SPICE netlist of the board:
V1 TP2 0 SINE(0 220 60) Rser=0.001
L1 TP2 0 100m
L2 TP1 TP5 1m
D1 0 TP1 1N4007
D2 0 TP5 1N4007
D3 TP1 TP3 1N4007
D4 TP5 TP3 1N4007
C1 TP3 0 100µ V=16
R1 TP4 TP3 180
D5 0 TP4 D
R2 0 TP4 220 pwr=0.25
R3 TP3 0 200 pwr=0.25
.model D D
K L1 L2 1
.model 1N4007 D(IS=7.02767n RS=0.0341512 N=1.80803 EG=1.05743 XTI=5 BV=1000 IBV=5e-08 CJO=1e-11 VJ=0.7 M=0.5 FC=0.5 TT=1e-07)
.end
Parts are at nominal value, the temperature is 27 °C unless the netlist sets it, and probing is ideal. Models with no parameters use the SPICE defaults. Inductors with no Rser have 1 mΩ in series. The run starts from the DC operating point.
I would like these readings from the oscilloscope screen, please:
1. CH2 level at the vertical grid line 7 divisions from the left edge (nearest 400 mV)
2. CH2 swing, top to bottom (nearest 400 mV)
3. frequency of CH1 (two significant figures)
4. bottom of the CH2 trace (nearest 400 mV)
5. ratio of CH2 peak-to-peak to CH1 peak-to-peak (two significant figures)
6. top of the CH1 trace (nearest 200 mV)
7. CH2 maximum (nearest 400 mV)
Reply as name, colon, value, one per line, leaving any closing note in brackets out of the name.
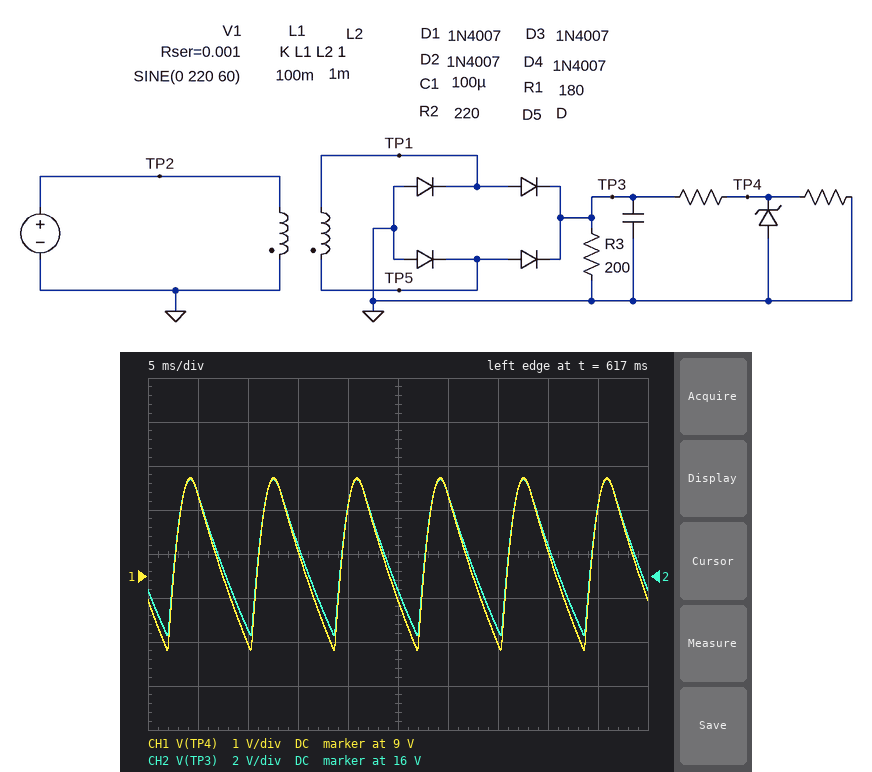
CH2 level at the vertical grid line 7 divisions from the left edge: 13.6 V
CH2 swing, top to bottom: 7.2 V
frequency of CH1: 120 Hz
bottom of the CH2 trace: 13.2 V
ratio of CH2 peak-to-peak to CH1 peak-to-peak: 1.8
top of the CH1 trace: 11.2 V
CH2 maximum: 20.4 V
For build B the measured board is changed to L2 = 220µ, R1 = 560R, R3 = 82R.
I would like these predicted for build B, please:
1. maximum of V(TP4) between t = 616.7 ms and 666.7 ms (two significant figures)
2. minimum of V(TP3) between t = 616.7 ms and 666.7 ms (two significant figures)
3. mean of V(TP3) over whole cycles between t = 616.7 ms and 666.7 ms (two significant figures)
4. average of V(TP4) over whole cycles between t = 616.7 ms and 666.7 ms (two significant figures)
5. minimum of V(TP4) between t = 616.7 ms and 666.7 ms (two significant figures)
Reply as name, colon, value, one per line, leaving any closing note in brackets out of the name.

maximum of V(TP4) between t = 616.7 ms and 666.7 ms: 2.5 V
minimum of V(TP3) between t = 616.7 ms and 666.7 ms: 4.4 V
mean of V(TP3) over whole cycles between t = 616.7 ms and 666.7 ms: 6.7 V
average of V(TP4) over whole cycles between t = 616.7 ms and 666.7 ms: 1.9 V
minimum of V(TP4) between t = 616.7 ms and 666.7 ms: 1.2 V
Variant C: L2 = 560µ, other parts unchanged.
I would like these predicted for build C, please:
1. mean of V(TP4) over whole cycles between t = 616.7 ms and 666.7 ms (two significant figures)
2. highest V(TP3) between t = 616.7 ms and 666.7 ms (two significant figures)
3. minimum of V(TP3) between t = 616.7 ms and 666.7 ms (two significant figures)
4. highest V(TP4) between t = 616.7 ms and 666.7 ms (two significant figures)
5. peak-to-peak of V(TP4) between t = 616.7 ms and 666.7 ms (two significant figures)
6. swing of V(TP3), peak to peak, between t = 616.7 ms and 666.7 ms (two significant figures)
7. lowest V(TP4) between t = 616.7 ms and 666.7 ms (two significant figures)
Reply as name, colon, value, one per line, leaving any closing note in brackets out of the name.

mean of V(TP4) over whole cycles between t = 616.7 ms and 666.7 ms: 6.9 V
highest V(TP3) between t = 616.7 ms and 666.7 ms: 15 V
minimum of V(TP3) between t = 616.7 ms and 666.7 ms: 9.7 V
highest V(TP4) between t = 616.7 ms and 666.7 ms: 8.2 V
peak-to-peak of V(TP4) between t = 616.7 ms and 666.7 ms: 2.9 V
swing of V(TP3), peak to peak, between t = 616.7 ms and 666.7 ms: 5.2 V
lowest V(TP4) between t = 616.7 ms and 666.7 ms: 5.3 V
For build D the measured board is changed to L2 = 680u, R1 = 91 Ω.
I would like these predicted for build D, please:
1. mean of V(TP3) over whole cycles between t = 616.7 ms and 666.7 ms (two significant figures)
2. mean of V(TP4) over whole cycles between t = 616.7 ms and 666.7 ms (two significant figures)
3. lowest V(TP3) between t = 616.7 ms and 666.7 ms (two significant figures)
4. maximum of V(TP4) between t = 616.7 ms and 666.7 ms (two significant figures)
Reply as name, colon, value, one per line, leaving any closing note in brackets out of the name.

mean of V(TP3) over whole cycles between t = 616.7 ms and 666.7 ms: 14 V
mean of V(TP4) over whole cycles between t = 616.7 ms and 666.7 ms: 9.7 V
lowest V(TP3) between t = 616.7 ms and 666.7 ms: 10 V
maximum of V(TP4) between t = 616.7 ms and 666.7 ms: 12 V
